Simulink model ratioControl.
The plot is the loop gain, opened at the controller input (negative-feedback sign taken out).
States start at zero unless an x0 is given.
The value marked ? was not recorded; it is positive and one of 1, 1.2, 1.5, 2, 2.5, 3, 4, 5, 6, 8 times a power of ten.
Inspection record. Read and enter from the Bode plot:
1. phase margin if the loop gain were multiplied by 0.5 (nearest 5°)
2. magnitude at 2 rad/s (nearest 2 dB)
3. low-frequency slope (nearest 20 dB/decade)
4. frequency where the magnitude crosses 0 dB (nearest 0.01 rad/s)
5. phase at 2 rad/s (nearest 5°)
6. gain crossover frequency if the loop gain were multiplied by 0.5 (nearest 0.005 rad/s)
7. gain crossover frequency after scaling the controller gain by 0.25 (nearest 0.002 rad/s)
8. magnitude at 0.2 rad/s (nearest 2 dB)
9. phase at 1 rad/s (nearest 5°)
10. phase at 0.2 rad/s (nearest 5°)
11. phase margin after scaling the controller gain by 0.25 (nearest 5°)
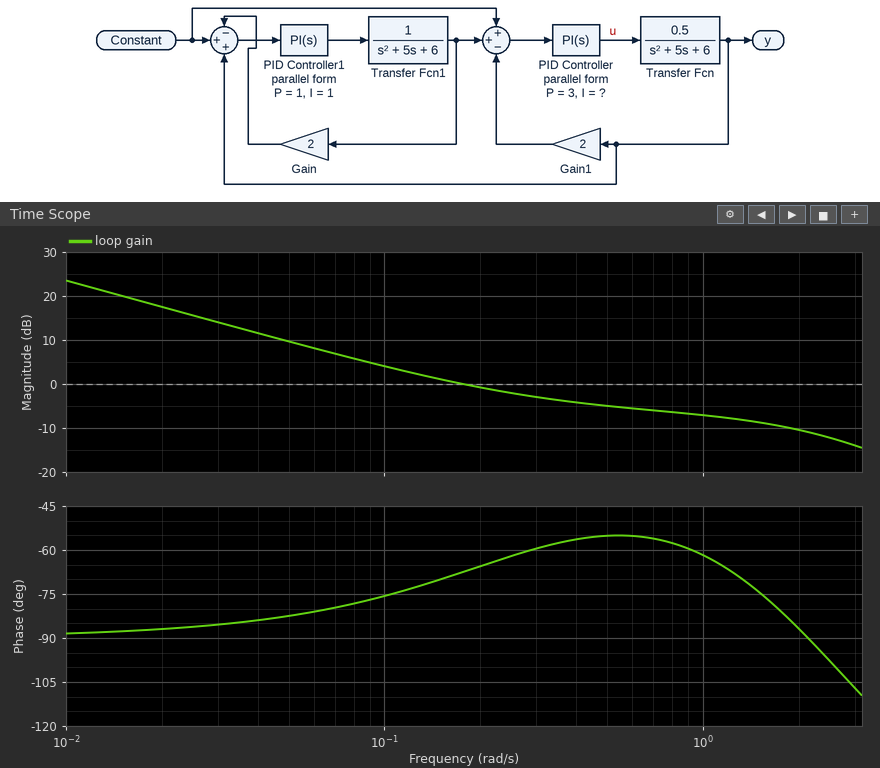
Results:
100°
-10 dB
-20 dB/decade
0.18 rad/s
-85°
0.080 rad/s
0.038 rad/s
0 dB
-60°
-65°
95°
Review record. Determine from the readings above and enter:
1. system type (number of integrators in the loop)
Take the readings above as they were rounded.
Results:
1
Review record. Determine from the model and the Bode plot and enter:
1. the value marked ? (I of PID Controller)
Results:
1.2
